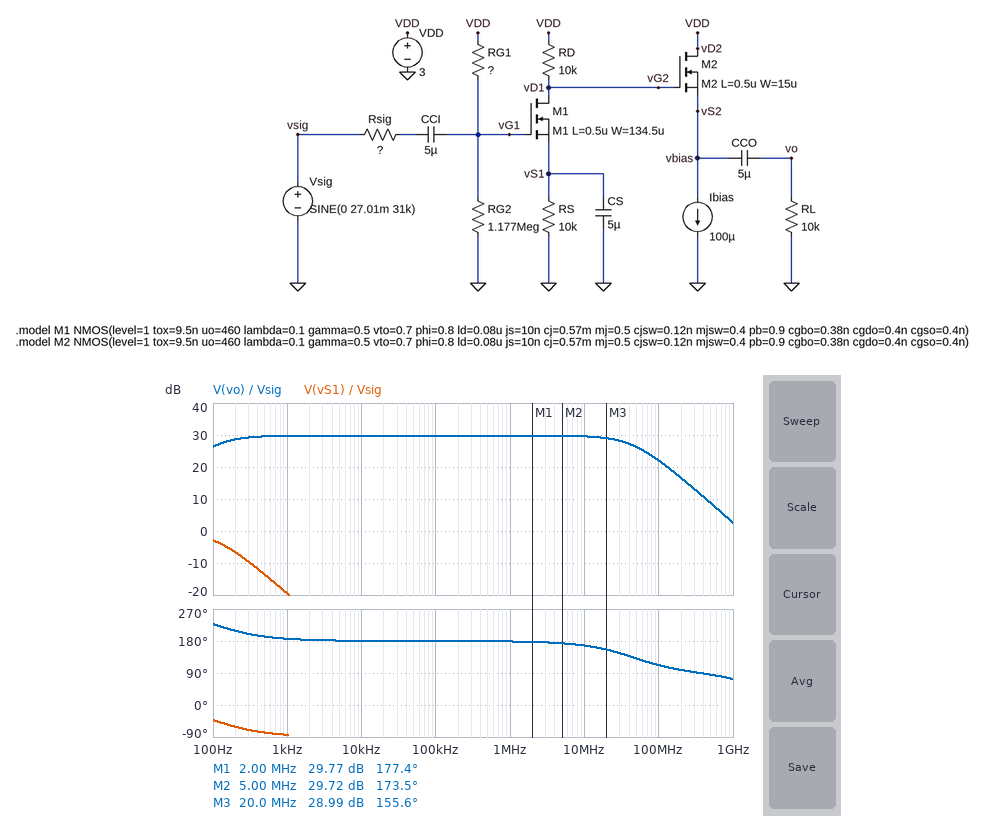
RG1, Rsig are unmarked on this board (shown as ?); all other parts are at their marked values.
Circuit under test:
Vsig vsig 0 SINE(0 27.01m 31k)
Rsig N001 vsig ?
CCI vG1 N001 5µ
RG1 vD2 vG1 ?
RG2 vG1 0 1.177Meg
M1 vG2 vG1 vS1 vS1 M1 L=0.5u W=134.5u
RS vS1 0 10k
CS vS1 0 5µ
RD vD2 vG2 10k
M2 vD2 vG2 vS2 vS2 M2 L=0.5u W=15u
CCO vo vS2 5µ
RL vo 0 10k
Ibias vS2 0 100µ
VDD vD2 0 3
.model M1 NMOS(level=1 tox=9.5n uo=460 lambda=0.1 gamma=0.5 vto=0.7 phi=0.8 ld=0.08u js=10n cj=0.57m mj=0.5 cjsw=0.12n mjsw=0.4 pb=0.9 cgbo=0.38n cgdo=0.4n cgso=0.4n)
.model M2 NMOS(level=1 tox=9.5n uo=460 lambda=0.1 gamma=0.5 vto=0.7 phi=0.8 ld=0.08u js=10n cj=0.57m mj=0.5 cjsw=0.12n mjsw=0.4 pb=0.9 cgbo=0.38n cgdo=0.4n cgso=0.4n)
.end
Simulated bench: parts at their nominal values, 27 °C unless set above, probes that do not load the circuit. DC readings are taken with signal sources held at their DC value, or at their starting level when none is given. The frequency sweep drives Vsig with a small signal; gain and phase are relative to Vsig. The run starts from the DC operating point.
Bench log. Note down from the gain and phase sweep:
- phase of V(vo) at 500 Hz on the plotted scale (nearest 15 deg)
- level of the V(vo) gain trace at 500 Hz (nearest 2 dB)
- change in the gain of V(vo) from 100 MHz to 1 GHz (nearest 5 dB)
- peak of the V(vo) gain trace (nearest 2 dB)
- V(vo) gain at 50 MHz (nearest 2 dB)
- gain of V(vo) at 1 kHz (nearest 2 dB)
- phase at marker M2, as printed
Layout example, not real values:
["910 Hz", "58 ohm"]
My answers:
["195 deg", "30 dB", "-20 dB", "30 dB", "26 dB", "30 dB", "173.5 deg"]
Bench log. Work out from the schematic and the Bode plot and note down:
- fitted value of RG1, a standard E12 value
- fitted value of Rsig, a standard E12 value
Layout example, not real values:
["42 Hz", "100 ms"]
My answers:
["1 MΩ", "1.5 kΩ"]
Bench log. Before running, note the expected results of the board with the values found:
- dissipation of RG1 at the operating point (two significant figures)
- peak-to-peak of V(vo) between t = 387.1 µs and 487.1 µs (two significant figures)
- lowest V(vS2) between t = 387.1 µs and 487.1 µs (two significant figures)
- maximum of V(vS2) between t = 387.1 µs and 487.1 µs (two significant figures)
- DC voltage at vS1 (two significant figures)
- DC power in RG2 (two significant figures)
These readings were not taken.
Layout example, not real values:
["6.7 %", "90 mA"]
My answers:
["1.9 µW", "1.6 V", "370 mV", "1.9 V", "870 mV", "2.2 µW"]
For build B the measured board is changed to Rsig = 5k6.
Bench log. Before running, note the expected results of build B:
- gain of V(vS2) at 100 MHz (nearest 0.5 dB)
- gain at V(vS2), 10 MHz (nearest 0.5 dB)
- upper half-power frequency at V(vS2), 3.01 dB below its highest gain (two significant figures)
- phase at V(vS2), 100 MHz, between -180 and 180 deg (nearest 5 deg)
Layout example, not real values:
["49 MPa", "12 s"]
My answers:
["12.5 dB", "28.0 dB", "14 MHz", "95 deg"]
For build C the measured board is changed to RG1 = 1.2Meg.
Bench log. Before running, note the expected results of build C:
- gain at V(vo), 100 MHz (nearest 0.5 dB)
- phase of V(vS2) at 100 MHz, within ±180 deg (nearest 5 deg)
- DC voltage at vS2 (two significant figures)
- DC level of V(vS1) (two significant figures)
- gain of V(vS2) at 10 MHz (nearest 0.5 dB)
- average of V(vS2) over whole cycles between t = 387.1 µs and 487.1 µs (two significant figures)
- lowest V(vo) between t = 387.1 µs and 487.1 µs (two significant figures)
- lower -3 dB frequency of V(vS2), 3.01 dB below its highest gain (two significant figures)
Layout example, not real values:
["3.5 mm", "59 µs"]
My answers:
["22.0 dB", "115 deg", "1.4 V", "740 mV", "29.0 dB", "1.3 V", "-880 mV", "100 Hz"]
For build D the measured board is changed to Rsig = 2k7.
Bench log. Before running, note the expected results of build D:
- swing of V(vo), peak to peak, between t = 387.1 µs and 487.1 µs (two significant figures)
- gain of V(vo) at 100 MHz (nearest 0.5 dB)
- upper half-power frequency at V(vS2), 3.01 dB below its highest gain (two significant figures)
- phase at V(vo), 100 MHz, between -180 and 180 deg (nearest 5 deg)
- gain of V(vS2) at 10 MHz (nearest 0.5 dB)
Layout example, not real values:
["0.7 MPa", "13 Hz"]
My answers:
["1.6 V", "18.0 dB", "27 MHz", "105 deg", "29.0 dB"]
